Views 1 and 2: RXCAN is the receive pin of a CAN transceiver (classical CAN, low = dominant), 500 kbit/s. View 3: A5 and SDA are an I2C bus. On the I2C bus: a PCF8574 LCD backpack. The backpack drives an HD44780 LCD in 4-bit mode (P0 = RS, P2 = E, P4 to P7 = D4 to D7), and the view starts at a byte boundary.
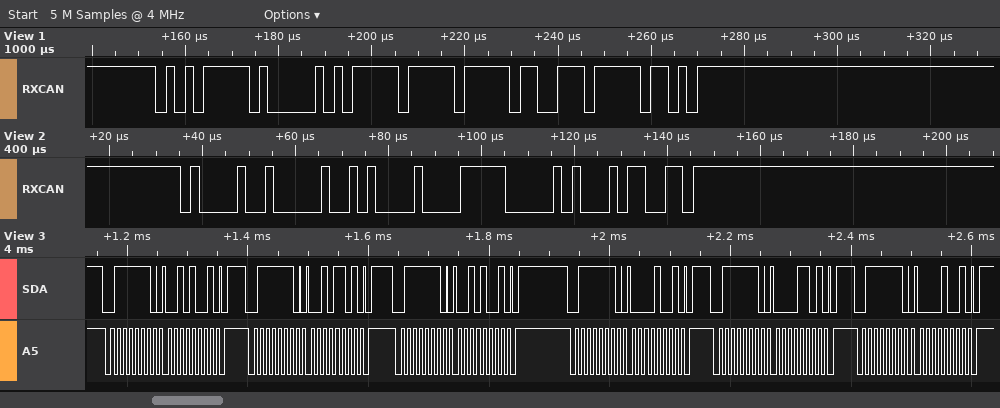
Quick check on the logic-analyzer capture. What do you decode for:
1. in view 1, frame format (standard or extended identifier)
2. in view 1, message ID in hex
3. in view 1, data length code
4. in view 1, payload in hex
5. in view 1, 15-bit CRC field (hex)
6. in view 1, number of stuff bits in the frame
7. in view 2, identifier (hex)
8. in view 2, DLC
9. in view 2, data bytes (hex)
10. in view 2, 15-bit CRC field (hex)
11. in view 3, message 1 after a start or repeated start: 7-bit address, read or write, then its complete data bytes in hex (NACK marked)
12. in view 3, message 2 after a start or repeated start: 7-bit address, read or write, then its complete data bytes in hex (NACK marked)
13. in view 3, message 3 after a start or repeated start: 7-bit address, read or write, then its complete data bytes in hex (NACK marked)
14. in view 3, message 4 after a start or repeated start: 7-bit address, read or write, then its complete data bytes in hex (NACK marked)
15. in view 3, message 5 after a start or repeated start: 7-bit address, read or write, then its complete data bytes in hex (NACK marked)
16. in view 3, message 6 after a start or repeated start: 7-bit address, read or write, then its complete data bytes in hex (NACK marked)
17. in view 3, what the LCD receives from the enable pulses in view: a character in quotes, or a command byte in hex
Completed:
standard
0x57E
2
FF FF
0x4EFE
6
0x424
2
84 3E
0x0459
0x3F write: 29
0x3F write: 2D
0x3F write: 29
0x3F write: 09
0x3F write: 0D
0x3F write: 09
' '
